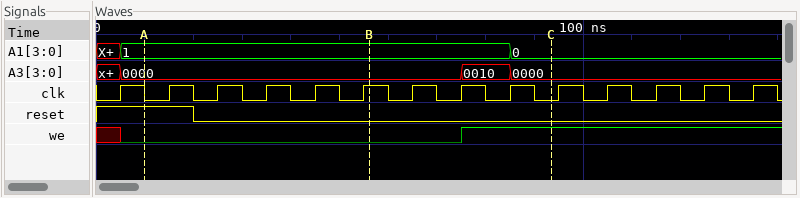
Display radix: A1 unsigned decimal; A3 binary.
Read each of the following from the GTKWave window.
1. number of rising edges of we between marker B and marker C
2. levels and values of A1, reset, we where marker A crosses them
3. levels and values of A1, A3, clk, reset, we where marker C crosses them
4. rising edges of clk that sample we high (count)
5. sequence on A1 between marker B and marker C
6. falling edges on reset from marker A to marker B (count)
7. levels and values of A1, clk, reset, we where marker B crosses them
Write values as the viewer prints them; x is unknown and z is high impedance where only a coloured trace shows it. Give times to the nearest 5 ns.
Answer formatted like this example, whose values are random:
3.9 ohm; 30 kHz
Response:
1; A1=1, reset=1, we=0; A1=0, A3=0000, clk=0, reset=0, we=1; 6; 1, 0; 1; A1=1, clk=1, reset=0, we=0
